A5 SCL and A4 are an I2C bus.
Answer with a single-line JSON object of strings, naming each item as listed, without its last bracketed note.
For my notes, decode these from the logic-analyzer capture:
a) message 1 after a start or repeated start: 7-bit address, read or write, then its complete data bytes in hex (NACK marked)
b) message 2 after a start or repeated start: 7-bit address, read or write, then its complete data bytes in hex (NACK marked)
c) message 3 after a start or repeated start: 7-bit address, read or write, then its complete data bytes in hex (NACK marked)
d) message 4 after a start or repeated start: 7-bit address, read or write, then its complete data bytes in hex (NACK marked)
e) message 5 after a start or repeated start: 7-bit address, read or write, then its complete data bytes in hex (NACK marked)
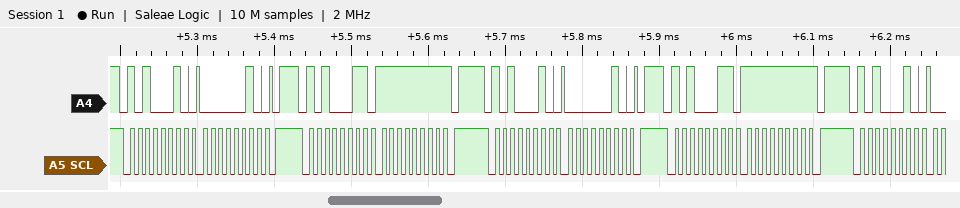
{"message 1 after a start or repeated start: 7-bit address, read or write, then its complete data bytes in hex": "0x51 write: 02", "message 2 after a start or repeated start: 7-bit address, read or write, then its complete data bytes in hex": "0x51 read: FF NACK", "message 3 after a start or repeated start: 7-bit address, read or write, then its complete data bytes in hex": "0x51 write: 02", "message 4 after a start or repeated start: 7-bit address, read or write, then its complete data bytes in hex": "0x51 read: FF NACK", "message 5 after a start or repeated start: 7-bit address, read or write, then its complete data bytes in hex": "0x51 write"}
